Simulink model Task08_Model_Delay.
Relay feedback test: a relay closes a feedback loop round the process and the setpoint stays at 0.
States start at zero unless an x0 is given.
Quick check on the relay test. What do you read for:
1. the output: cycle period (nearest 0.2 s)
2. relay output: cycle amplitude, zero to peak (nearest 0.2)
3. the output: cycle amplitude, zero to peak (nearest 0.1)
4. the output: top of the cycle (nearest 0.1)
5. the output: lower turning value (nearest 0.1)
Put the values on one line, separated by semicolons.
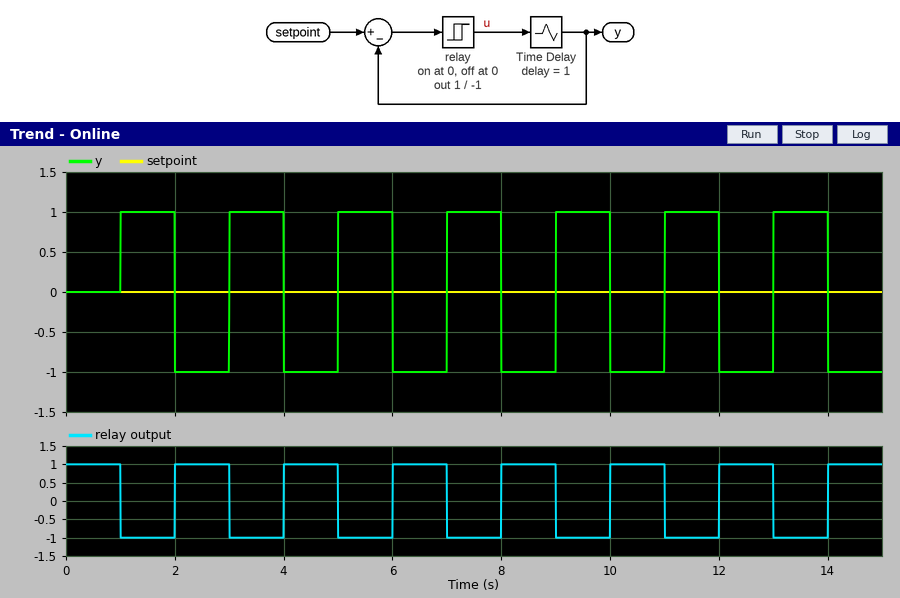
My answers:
2.0 s; 1.0; 1.0; 1.0; -1.0
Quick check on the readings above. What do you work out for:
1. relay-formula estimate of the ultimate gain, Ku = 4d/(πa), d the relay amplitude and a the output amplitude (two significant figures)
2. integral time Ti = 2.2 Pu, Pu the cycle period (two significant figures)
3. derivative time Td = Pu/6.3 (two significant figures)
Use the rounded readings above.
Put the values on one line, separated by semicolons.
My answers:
1.3; 4.4 s; 0.32 s
